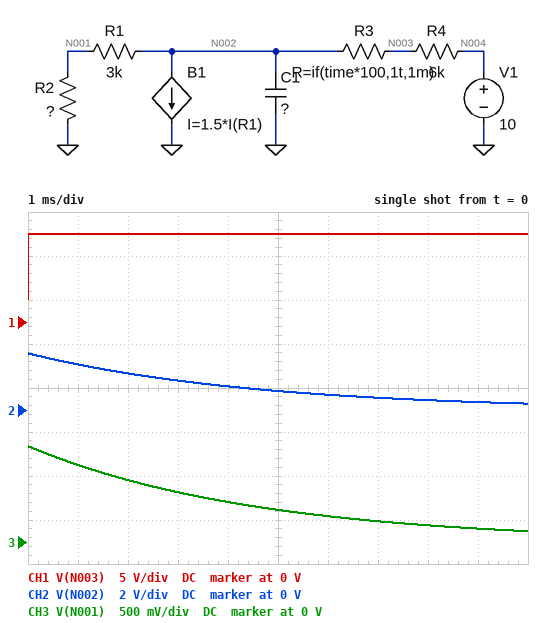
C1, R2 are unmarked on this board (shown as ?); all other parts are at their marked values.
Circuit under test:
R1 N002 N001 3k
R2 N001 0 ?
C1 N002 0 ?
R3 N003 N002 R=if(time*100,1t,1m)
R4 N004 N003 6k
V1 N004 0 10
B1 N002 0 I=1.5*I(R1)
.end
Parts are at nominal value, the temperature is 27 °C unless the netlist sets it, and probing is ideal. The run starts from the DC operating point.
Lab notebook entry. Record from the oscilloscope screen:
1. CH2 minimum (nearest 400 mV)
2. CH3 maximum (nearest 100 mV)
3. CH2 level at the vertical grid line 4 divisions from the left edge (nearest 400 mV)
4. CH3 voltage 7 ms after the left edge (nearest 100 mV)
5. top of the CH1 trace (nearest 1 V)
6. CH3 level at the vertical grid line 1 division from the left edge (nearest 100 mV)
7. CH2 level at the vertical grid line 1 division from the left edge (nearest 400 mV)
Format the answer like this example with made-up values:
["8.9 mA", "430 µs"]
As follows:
["400 mV", "1.1 V", "1.2 V", "200 mV", "10 V", "900 mV", "2.0 V"]
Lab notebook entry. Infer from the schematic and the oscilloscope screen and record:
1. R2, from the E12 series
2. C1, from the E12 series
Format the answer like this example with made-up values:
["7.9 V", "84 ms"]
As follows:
["2.2 kΩ", "2.2 µF"]
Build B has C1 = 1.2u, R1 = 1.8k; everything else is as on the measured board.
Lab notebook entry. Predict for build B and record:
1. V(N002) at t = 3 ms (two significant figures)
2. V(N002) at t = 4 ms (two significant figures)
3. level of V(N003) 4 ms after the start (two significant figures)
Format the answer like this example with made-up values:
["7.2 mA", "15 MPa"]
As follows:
["440 mV", "260 mV", "10 V"]
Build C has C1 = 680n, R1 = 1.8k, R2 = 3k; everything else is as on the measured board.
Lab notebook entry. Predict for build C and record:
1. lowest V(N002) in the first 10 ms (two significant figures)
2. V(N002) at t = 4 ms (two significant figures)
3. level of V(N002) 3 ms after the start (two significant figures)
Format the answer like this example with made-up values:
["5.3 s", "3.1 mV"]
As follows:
["1.1 mV", "110 mV", "240 mV"]
